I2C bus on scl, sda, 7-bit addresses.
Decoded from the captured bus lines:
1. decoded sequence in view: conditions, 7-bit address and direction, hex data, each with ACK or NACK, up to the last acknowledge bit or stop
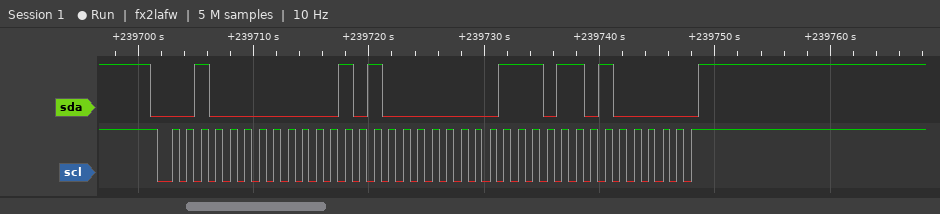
start, address 10 write ACK, 14 ACK, 07 ACK, D0 ACK, stop
